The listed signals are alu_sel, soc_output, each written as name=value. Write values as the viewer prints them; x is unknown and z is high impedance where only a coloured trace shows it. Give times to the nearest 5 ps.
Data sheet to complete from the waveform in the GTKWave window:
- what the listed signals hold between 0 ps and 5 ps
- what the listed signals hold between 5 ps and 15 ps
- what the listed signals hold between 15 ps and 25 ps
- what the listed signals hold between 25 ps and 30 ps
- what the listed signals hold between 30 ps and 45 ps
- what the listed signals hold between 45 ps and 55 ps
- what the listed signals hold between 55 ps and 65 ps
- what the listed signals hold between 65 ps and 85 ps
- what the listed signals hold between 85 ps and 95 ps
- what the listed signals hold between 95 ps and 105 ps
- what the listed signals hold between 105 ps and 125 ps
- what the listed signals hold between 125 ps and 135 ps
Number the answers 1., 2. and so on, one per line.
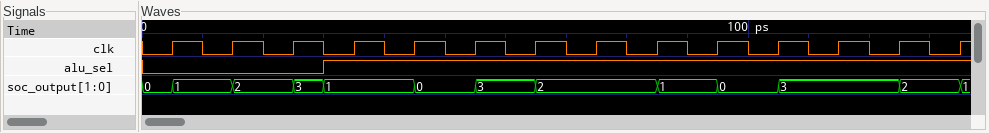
1. alu_sel=0, soc_output=0
2. alu_sel=0, soc_output=1
3. alu_sel=0, soc_output=2
4. alu_sel=0, soc_output=3
5. alu_sel=1, soc_output=1
6. alu_sel=1, soc_output=0
7. alu_sel=1, soc_output=3
8. alu_sel=1, soc_output=2
9. alu_sel=1, soc_output=1
10. alu_sel=1, soc_output=0
11. alu_sel=1, soc_output=3
12. alu_sel=1, soc_output=2
